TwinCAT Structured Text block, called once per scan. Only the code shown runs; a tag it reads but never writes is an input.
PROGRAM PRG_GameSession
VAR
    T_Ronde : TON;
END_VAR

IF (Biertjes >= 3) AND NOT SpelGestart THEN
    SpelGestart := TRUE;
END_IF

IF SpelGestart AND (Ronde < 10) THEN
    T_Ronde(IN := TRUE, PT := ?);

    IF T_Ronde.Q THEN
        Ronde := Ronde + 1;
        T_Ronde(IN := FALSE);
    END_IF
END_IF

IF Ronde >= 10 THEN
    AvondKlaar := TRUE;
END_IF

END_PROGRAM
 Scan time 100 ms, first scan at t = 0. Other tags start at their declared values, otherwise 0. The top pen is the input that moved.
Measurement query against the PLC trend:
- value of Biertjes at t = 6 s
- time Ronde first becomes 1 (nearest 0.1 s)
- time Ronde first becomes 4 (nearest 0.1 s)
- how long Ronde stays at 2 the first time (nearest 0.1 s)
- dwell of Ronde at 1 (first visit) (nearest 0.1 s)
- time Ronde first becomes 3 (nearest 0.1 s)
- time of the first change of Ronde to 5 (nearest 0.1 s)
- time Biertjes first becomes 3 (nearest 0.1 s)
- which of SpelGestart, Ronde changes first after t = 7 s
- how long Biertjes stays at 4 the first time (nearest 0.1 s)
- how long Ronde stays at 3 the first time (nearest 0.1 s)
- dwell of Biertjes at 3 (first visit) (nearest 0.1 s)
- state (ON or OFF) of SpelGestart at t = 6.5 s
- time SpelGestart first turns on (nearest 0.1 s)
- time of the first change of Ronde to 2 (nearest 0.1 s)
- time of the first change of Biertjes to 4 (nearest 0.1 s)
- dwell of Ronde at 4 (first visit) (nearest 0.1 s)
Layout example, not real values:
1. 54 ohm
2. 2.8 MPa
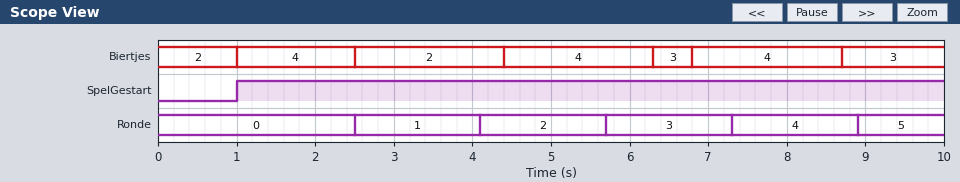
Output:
1. 4
2. 2.5 s
3. 7.3 s
4. 1.6 s
5. 1.6 s
6. 5.7 s
7. 8.9 s
8. 6.3 s
9. Ronde
10. 1.5 s
11. 1.6 s
12. 0.5 s
13. ON
14. 1.0 s
15. 4.1 s
16. 1.0 s
17. 1.6 s
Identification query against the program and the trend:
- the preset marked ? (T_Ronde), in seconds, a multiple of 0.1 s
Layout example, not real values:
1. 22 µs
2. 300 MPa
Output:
1. 1.5 s
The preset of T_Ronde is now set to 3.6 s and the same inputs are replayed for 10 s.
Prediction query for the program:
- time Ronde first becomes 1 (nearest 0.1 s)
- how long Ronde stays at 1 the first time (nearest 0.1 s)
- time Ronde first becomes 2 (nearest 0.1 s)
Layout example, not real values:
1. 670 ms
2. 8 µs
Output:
1. 4.6 s
2. 3.7 s
3. 8.3 s
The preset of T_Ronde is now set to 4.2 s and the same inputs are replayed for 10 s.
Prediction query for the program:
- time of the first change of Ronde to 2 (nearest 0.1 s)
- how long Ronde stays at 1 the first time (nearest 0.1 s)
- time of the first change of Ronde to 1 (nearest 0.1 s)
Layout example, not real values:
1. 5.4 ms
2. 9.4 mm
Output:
1. 9.5 s
2. 4.3 s
3. 5.2 s
